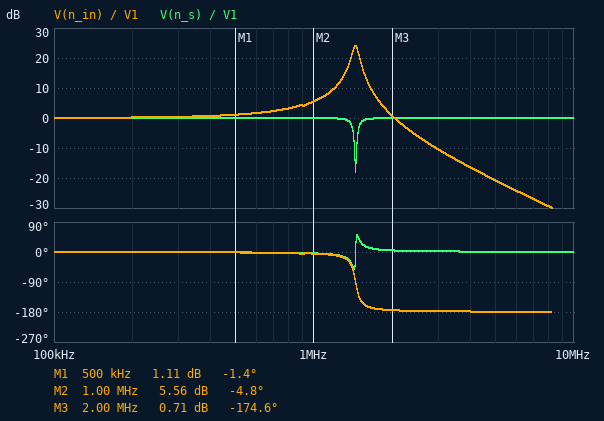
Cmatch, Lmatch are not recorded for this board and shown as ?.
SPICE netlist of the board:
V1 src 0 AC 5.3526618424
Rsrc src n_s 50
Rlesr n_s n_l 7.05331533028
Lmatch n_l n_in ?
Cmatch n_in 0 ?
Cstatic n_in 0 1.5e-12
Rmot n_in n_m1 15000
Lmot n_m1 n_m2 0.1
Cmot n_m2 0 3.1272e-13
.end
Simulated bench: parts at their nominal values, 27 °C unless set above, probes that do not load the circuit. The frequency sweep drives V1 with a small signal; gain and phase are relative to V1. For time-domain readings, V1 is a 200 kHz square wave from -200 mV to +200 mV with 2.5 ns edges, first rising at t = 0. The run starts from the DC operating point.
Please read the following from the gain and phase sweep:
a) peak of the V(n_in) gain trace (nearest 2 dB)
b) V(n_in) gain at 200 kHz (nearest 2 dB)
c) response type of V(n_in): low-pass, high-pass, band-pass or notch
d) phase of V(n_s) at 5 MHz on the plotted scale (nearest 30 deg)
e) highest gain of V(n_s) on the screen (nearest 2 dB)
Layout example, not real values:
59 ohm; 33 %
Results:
24 dB; 0 dB; band-pass; 0 deg; 0 dB
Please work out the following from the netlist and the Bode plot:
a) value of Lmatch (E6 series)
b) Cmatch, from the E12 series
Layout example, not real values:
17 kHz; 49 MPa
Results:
100 µH; 120 pF
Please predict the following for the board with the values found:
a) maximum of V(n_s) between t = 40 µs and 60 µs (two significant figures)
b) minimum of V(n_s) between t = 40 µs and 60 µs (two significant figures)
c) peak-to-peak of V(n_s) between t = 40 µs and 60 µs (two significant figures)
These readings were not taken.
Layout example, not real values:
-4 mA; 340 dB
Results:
230 mV; -230 mV; 460 mV
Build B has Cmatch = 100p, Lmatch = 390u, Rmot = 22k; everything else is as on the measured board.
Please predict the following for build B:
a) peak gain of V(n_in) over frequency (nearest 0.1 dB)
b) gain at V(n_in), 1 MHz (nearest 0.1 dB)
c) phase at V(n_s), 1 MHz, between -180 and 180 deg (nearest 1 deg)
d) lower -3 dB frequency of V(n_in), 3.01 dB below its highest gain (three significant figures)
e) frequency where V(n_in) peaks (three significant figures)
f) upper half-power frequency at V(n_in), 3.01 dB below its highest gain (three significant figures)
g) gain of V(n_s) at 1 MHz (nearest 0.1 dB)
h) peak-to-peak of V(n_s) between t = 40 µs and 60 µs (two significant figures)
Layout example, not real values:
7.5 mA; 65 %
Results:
30.1 dB; 5.3 dB; 3 deg; 782 kHz; 794 kHz; 806 kHz; 0 dB; 410 mV
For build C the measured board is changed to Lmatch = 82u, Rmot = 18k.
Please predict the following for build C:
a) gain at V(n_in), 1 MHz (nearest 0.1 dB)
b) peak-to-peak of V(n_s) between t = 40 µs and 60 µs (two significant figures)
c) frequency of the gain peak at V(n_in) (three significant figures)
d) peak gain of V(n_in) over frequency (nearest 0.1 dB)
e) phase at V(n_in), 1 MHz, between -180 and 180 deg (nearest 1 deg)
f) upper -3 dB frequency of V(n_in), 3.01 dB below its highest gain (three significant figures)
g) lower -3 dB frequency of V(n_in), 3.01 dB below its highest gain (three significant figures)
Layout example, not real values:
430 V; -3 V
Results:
4.3 dB; 430 mV; 1.59 MHz; 23.2 dB; -4 deg; 1.65 MHz; 1.54 MHz
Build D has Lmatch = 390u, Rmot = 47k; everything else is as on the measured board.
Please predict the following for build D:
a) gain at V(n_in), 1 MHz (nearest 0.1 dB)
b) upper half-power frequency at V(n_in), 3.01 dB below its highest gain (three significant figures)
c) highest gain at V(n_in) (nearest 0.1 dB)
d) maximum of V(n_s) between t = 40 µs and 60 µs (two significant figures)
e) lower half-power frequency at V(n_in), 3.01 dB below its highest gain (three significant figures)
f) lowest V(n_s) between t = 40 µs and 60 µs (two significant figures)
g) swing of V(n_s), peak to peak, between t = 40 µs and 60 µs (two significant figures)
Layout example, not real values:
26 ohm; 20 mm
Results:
1.4 dB; 740 kHz; 29.5 dB; 210 mV; 716 kHz; -210 mV; 410 mV
